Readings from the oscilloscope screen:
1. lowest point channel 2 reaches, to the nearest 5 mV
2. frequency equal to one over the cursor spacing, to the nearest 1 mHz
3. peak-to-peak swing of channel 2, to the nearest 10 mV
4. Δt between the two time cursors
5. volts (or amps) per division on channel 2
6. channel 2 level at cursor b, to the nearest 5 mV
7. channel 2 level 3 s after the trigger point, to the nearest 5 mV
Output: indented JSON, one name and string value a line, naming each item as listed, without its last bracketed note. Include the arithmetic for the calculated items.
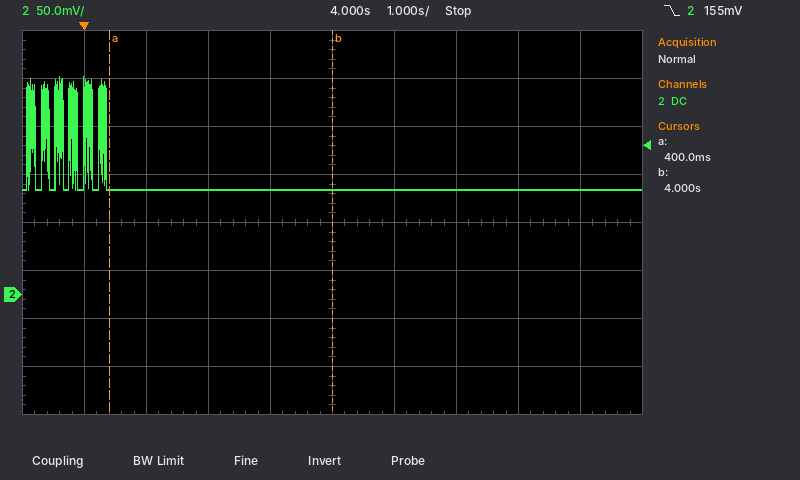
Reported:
{
  "lowest point channel 2 reaches, to the nearest 5 mV": "110 mV",
  "frequency equal to one over the cursor spacing, to the nearest 1 mHz": "1 / 3.6 s ≈ 278 mHz",
  "peak-to-peak swing of channel 2, to the nearest 10 mV": "120 mV",
  "Δt between the two time cursors": "4 s − (400 ms) = 3.6 s",
  "volts (or amps) per division on channel 2": "50 mV",
  "channel 2 level at cursor b, to the nearest 5 mV": "110 mV",
  "channel 2 level 3 s after the trigger point, to the nearest 5 mV": "110 mV"
}
